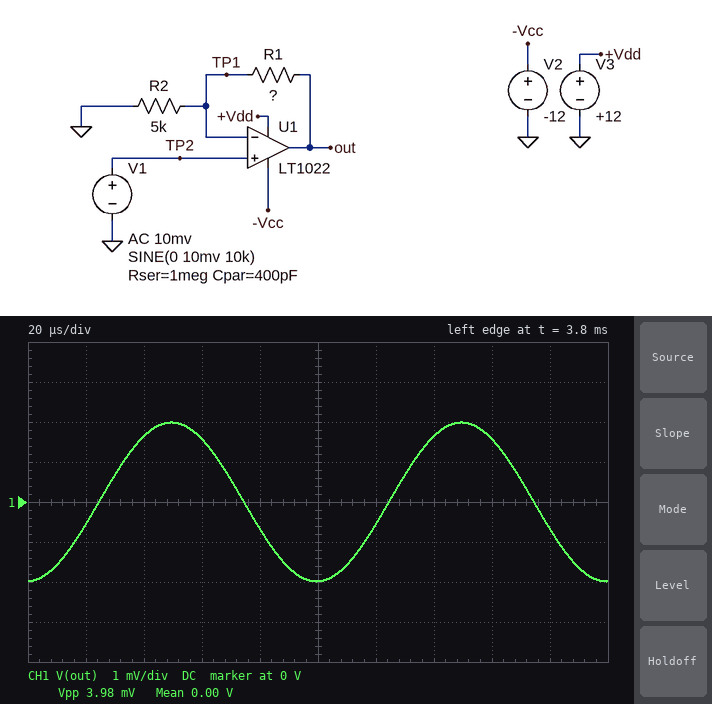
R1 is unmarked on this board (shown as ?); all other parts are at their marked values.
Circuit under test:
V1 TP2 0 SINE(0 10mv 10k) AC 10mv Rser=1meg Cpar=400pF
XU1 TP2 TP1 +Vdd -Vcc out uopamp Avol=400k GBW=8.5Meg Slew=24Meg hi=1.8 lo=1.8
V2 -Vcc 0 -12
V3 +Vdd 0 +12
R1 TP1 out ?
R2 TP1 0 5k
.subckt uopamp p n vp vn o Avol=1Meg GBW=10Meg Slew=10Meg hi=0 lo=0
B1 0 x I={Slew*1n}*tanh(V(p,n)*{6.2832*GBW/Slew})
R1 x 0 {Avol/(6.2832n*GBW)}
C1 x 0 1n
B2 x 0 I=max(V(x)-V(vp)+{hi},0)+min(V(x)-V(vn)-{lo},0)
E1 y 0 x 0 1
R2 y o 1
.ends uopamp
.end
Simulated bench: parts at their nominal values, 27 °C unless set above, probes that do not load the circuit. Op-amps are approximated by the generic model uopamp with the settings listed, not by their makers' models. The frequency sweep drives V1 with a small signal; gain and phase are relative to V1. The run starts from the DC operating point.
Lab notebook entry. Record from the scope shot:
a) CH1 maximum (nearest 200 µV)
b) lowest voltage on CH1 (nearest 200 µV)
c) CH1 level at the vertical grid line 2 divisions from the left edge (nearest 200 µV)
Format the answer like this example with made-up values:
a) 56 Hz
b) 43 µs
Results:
a) 2.0 mV
b) -2.0 mV
c) 1.6 mV
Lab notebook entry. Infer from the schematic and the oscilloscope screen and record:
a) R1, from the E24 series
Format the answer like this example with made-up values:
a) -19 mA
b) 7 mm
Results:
a) 20 kΩ
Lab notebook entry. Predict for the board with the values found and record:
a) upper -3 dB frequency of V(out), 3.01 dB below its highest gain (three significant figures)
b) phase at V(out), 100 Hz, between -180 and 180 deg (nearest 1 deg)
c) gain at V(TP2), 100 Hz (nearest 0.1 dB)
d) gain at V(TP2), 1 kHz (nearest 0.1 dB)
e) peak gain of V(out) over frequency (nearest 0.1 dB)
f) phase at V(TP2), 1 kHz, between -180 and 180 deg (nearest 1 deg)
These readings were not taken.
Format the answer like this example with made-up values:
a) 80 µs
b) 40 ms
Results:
a) 398 Hz
b) -14 deg
c) -0.3 dB
d) -8.6 dB
e) 14.0 dB
f) -68 deg
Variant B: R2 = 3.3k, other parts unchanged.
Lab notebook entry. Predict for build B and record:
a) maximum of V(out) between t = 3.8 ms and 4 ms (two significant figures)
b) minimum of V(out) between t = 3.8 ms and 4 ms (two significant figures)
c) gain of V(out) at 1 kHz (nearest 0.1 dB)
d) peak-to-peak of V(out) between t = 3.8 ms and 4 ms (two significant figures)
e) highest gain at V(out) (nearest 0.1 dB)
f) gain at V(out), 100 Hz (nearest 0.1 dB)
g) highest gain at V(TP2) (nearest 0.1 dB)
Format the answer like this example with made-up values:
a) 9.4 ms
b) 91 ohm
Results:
a) 2.8 mV
b) -2.8 mV
c) 8.3 dB
d) 5.6 mV
e) 17.0 dB
f) 16.7 dB
g) 0 dB
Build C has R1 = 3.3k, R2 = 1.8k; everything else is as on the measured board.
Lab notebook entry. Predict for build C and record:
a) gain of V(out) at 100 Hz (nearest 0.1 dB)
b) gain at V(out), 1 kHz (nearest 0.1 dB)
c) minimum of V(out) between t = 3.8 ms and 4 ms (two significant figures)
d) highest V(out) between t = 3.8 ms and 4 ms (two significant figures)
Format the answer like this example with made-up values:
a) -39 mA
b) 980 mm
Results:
a) 8.8 dB
b) 0.4 dB
c) -1.1 mV
d) 1.1 mV
